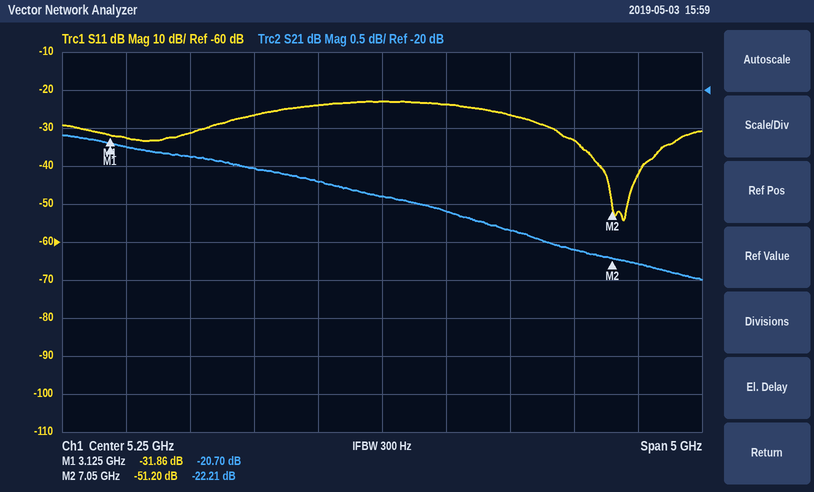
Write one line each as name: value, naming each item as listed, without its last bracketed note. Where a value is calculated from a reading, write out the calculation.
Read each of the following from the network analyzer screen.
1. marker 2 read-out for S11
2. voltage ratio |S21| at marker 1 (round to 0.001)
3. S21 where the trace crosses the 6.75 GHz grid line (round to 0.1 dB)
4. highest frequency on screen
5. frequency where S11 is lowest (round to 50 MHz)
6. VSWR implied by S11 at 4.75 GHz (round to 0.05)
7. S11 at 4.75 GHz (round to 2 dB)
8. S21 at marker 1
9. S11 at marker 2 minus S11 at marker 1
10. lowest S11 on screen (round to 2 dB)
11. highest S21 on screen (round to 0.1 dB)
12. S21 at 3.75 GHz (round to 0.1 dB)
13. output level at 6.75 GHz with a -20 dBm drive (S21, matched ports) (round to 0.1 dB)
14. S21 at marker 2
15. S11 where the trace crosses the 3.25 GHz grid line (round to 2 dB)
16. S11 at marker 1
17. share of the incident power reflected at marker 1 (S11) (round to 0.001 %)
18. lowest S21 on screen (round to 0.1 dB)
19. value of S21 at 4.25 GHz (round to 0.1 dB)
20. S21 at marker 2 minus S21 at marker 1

marker 2 read-out for S11: -51.20 dB
voltage ratio |S21| at marker 1: 10^(-20.7/20) ≈ 0.092
S21 where the trace crosses the 6.75 GHz grid line: -22.1 dB
highest frequency on screen: 7.75 GHz
frequency where S11 is lowest: 7.15 GHz
VSWR implied by S11 at 4.75 GHz: |Γ| = 10^(-24/20) = 0.0631; VSWR = (1 + 0.0631)/(1 − 0.0631) ≈ 1.13, so 1.15 to the nearest 0.05
S11 at 4.75 GHz: -24 dB
S21 at marker 1: -20.70 dB
S11 at marker 2 minus S11 at marker 1: -51.2 − (-31.86) = -19.34 dB
lowest S11 on screen: -54 dB
highest S21 on screen: -20.6 dB
S21 at 3.75 GHz: -20.9 dB
output level at 6.75 GHz with a -20 dBm drive (S21, matched ports): -20 dBm + (-22.1 dB) = -42.1 dBm
S21 at marker 2: -22.21 dB
S11 where the trace crosses the 3.25 GHz grid line: -32 dB
S11 at marker 1: -31.86 dB
share of the incident power reflected at marker 1 (S11): 10^(-31.86/10) ≈ 0.065 %
lowest S21 on screen: -22.5 dB
value of S21 at 4.25 GHz: -21.0 dB
S21 at marker 2 minus S21 at marker 1: -22.21 − (-20.7) = -1.51 dB
